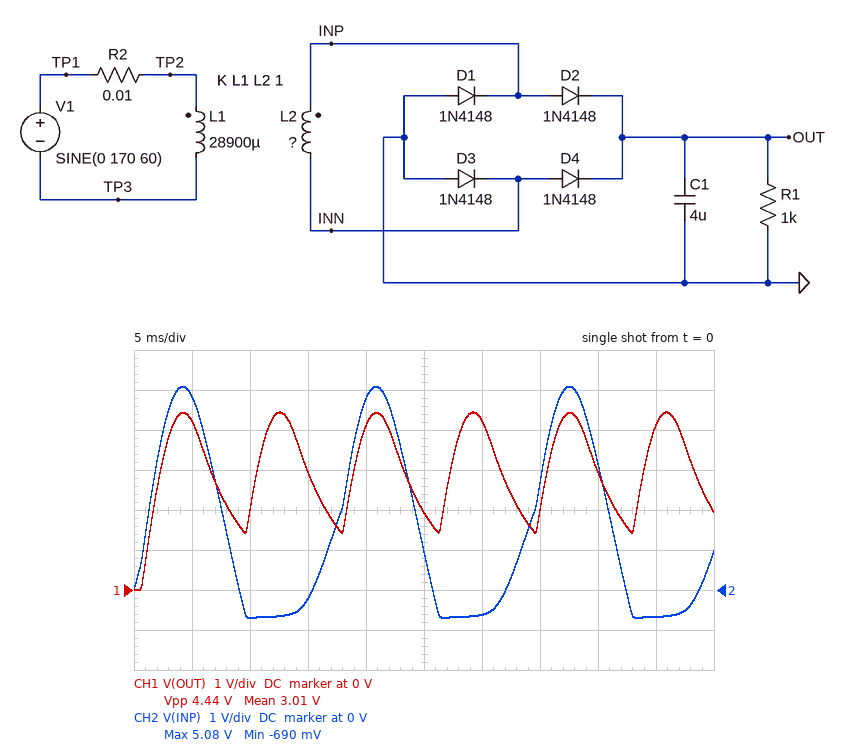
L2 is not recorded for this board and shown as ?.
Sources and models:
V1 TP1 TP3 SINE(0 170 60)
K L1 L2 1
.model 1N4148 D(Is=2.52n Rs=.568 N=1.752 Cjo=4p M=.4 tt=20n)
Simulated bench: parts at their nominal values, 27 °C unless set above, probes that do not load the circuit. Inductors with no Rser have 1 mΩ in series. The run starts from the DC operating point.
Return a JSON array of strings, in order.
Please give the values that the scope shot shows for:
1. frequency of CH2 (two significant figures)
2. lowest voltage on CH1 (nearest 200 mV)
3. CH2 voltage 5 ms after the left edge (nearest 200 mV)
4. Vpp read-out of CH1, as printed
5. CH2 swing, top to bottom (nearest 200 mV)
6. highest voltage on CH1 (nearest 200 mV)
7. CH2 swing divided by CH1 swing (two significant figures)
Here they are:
["60 Hz", "0 V", "4.8 V", "4.44 V", "5.8 V", "4.4 V", "1.3"]
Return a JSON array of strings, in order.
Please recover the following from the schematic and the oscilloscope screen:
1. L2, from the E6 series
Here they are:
["33 µH"]
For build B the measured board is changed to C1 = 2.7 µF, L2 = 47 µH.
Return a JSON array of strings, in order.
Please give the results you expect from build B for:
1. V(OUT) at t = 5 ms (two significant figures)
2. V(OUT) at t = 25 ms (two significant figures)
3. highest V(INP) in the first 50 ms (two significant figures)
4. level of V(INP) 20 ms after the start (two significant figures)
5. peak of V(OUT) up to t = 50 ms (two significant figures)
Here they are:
["5.2 V", "1.8 V", "6.2 V", "5.8 V", "5.5 V"]
